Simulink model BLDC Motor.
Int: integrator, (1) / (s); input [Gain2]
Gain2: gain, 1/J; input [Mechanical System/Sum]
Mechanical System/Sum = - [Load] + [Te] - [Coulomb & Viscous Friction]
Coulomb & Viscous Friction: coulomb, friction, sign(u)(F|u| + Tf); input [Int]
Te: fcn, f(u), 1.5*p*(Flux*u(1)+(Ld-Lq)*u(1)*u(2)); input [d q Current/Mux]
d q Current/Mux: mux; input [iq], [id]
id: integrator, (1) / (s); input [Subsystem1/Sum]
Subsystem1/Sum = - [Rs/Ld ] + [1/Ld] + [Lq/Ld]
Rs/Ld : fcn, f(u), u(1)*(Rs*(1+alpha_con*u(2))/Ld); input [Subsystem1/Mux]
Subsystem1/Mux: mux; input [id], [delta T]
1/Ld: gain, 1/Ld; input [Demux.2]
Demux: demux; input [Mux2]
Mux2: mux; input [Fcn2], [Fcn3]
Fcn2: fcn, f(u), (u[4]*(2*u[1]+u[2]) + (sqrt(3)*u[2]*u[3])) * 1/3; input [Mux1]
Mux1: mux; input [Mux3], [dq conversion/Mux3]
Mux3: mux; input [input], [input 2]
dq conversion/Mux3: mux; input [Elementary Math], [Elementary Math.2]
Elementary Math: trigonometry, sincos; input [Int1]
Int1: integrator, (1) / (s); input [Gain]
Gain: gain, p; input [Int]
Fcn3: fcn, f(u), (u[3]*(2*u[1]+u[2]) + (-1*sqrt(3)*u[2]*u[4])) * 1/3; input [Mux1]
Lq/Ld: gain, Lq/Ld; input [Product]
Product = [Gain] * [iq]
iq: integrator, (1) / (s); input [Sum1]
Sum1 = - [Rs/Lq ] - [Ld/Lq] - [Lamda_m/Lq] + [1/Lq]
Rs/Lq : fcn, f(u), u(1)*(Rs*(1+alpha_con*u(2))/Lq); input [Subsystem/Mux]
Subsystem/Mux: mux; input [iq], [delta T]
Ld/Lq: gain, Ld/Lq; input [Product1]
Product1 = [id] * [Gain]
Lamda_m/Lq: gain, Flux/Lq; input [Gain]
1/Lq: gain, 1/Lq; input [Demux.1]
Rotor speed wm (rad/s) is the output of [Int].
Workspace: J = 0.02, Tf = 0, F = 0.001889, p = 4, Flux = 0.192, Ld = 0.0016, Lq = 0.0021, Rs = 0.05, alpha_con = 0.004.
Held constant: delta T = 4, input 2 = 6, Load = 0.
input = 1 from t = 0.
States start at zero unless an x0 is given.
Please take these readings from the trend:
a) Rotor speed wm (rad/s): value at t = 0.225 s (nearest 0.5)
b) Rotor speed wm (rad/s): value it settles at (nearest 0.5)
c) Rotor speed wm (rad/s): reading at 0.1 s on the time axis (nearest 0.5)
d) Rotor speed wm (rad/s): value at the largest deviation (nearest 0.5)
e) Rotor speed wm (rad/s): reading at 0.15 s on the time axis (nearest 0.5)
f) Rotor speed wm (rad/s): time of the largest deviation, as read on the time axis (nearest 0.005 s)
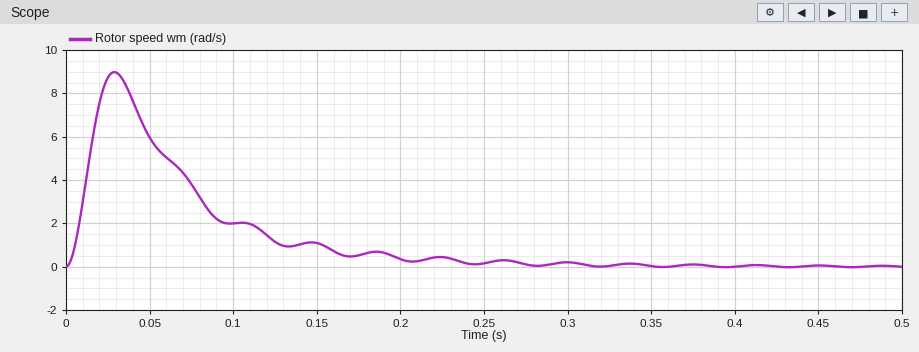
0.5
0.0
2.0
9.0
1.0
0.030 s
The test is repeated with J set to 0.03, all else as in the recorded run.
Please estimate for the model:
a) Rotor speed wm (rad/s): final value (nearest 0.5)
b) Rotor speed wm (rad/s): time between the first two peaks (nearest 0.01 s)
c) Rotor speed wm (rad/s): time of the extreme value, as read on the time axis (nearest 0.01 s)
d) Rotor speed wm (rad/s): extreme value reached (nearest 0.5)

0.0
0.11 s
0.04 s
9.5
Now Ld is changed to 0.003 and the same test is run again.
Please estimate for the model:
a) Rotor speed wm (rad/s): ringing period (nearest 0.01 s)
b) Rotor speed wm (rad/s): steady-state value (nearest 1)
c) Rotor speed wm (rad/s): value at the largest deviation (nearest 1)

0.09 s
0
10
